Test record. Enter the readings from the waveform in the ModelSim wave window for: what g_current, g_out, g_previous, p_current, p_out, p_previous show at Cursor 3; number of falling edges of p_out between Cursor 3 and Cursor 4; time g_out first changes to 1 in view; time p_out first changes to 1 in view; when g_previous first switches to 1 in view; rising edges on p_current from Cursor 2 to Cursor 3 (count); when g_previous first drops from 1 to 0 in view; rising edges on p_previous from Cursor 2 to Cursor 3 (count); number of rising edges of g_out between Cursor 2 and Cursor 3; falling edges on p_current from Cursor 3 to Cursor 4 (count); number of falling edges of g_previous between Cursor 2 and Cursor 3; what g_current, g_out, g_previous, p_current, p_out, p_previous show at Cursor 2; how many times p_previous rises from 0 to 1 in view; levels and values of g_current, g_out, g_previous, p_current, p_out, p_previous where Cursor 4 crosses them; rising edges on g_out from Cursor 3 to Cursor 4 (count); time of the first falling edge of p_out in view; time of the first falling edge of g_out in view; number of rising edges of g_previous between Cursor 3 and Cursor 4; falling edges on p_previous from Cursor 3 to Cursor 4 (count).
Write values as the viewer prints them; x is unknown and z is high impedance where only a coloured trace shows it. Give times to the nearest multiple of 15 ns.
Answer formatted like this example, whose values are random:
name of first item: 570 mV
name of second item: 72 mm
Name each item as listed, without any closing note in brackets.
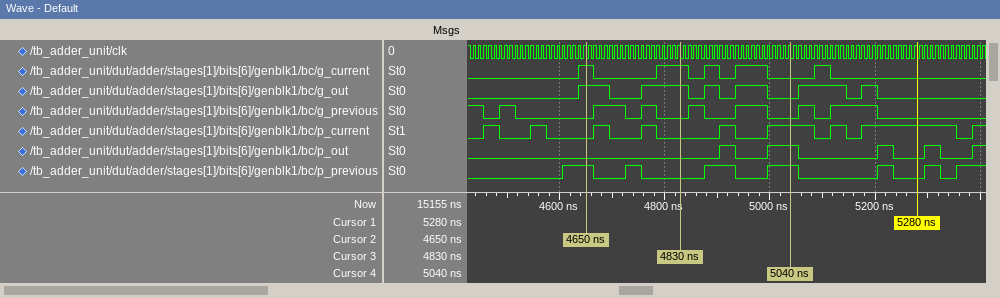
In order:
what g_current, g_out, g_previous, p_current, p_out, p_previous show at Cursor 3: g_current=1, g_out=1, g_previous=0, p_current=0, p_out=0, p_previous=0
number of falling edges of p_out between Cursor 3 and Cursor 4: 1
time g_out first changes to 1 in view: 4635 ns
time p_out first changes to 1 in view: 4905 ns
when g_previous first switches to 1 in view: 4485 ns
rising edges on p_current from Cursor 2 to Cursor 3: 2
when g_previous first drops from 1 to 0 in view: 4455 ns
rising edges on p_previous from Cursor 2 to Cursor 3: 1
number of rising edges of g_out between Cursor 2 and Cursor 3: 1
falling edges on p_current from Cursor 3 to Cursor 4: 1
number of falling edges of g_previous between Cursor 2 and Cursor 3: 2
what g_current, g_out, g_previous, p_current, p_out, p_previous show at Cursor 2: g_current=1, g_out=1, g_previous=0, p_current=0, p_out=0, p_previous=1
how many times p_previous rises from 0 to 1 in view: 7
levels and values of g_current, g_out, g_previous, p_current, p_out, p_previous where Cursor 4 crosses them: g_current=0, g_out=0, g_previous=0, p_current=1, p_out=1, p_previous=1
rising edges on g_out from Cursor 3 to Cursor 4: 2
time of the first falling edge of p_out in view: 4935 ns
time of the first falling edge of g_out in view: 4695 ns
number of rising edges of g_previous between Cursor 3 and Cursor 4: 2
falling edges on p_previous from Cursor 3 to Cursor 4: 1
